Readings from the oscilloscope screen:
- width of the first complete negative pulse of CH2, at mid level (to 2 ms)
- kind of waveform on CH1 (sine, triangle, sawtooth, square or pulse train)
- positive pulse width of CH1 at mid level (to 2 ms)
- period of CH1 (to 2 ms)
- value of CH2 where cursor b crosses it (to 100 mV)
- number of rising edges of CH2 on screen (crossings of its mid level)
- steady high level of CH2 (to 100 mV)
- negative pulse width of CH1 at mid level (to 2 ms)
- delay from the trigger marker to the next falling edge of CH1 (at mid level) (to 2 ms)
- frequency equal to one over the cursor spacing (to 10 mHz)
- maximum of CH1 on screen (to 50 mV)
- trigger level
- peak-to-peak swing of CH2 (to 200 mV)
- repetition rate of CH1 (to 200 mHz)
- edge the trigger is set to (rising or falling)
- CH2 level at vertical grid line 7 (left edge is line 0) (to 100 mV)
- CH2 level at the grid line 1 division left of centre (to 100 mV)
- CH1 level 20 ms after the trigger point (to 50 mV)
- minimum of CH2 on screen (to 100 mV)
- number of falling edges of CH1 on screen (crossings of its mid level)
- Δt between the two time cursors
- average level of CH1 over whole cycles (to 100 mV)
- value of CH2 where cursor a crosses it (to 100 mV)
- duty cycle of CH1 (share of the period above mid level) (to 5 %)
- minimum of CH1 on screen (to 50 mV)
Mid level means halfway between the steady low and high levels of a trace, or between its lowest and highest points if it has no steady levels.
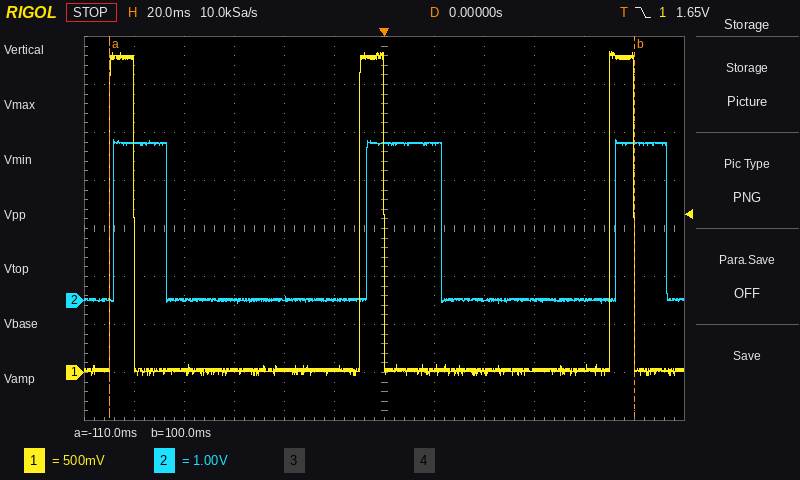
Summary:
80 ms
pulse train
10 ms
100 ms
3.3 V
3
3.3 V
90 ms
100 ms
4.76 Hz
3.35 V
1.65 V
3.4 V
10.0 Hz
falling
3.3 V
0.0 V
50 mV
-100 mV
3
210 ms
300 mV
0.0 V
10 %
-50 mV
